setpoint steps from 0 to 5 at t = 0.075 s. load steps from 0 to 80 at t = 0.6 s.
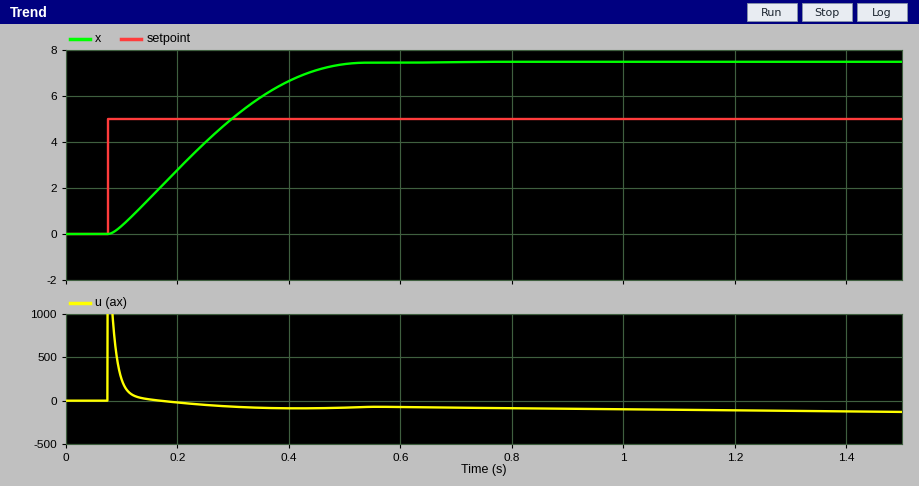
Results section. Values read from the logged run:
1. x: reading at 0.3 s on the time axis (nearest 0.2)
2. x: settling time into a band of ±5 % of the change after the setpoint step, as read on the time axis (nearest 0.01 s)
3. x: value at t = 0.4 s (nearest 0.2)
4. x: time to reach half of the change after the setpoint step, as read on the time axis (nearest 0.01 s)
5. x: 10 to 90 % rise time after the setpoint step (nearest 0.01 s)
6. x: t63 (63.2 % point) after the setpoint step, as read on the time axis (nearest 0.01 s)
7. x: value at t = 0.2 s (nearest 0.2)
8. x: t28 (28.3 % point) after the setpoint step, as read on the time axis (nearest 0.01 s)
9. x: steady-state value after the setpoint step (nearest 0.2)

5.0
0.44 s
6.6
0.24 s
0.29 s
0.28 s
2.8
0.17 s
7.4
